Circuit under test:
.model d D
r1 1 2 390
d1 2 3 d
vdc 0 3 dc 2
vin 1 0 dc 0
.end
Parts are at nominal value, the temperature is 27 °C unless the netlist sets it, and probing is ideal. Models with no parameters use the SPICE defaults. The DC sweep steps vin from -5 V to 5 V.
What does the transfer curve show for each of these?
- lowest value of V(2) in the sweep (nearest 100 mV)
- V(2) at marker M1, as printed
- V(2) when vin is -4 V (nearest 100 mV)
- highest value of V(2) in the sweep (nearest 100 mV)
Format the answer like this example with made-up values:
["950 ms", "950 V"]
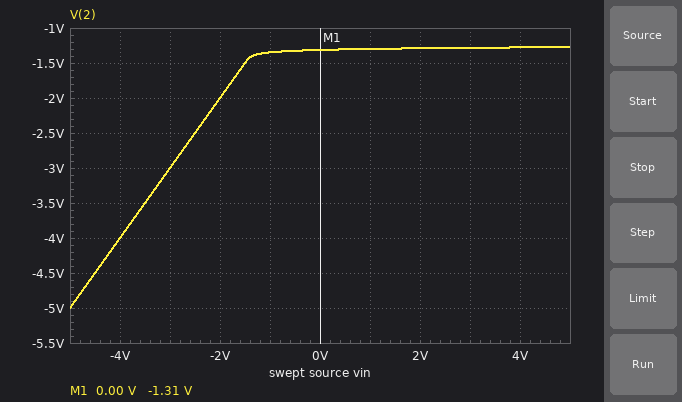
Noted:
["-5.0 V", "-1.31 V", "-4.0 V", "-1.3 V"]
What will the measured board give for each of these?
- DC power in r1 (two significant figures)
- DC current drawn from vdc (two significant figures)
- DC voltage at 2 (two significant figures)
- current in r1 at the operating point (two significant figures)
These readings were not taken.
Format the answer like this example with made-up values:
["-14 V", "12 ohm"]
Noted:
["4.4 mW", "3.4 mA", "-1.3 V", "3.4 mA"]
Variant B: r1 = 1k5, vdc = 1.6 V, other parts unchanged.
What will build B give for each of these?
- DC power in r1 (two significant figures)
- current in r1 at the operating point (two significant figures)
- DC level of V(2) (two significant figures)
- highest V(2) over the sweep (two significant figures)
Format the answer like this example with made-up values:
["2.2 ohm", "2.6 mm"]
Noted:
["610 µW", "640 µA", "-960 mV", "-910 mV"]
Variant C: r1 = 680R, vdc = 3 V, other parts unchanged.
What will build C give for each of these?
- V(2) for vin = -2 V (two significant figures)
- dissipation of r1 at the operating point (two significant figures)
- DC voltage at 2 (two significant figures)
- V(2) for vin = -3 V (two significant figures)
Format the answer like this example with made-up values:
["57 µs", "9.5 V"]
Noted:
["-2.4 V", "7.9 mW", "-2.3 V", "-3.0 V"]
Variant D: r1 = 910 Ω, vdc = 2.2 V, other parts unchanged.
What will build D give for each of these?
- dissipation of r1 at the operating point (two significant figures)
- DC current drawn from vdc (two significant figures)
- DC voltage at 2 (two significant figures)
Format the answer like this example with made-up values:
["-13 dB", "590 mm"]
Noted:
["2.6 mW", "1.7 mA", "-1.5 V"]
